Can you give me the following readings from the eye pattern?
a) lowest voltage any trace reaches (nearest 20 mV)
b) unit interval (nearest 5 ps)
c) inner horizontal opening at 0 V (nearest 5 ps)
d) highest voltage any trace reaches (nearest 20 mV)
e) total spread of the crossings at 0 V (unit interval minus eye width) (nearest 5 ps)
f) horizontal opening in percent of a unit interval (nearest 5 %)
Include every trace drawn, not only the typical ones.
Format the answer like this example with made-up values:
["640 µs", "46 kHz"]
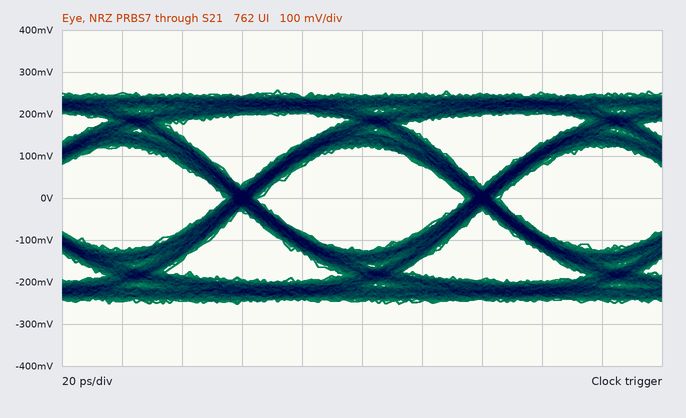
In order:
["-260 mV", "80 ps", "70 ps", "260 mV", "10 ps", "85 %"]
